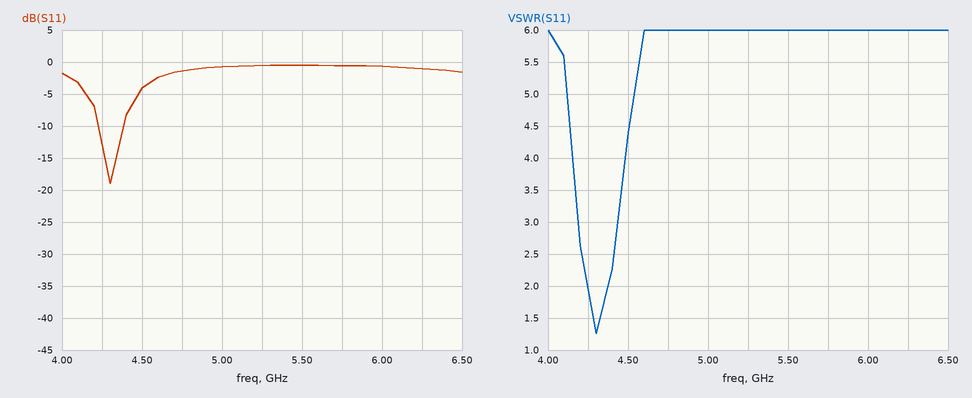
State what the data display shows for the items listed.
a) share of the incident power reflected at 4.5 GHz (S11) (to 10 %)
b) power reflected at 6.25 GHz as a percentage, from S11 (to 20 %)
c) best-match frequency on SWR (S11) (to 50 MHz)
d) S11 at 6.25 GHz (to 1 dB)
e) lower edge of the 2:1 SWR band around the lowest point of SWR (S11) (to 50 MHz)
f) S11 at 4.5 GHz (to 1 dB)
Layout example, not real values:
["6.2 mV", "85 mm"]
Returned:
["40 %", "80 %", "4.30 GHz", "-1 dB", "4.25 GHz", "-4 dB"]
